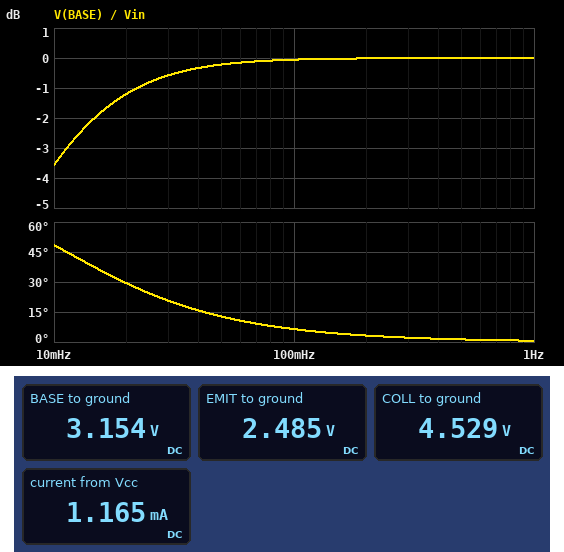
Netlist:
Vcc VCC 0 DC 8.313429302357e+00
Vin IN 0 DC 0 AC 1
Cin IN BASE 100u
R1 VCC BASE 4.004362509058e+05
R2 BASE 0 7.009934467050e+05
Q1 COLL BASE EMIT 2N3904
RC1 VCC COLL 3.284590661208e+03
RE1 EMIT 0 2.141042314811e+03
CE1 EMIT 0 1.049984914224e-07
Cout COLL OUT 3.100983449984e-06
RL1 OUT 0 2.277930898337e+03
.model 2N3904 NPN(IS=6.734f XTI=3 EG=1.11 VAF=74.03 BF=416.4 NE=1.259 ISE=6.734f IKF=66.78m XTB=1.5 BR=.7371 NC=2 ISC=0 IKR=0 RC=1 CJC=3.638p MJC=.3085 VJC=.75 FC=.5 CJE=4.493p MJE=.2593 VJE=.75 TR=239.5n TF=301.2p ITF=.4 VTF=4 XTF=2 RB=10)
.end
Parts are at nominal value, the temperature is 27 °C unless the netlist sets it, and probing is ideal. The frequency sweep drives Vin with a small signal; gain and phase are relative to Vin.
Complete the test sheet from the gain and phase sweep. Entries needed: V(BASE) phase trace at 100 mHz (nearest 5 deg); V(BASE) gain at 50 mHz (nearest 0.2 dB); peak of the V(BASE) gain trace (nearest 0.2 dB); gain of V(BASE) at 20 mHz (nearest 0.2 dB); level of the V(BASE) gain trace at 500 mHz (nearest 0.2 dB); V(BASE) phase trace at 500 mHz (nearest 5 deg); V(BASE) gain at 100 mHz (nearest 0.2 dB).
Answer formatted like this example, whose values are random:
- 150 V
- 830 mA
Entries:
- 5 deg
- -0.2 dB
- 0 dB
- -1.2 dB
- 0 dB
- 0 deg
- 0 dB
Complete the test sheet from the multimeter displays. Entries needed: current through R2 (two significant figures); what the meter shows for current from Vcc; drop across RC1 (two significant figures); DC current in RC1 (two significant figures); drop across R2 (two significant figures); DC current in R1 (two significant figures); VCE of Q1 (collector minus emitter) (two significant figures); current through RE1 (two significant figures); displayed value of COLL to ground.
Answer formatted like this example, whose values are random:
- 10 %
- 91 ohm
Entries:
- 4.5 µA
- 1.165 mA
- 3.8 V
- 1.2 mA
- 3.2 V
- 13 µA
- 2.0 V
- 1.2 mA
- 4.529 V
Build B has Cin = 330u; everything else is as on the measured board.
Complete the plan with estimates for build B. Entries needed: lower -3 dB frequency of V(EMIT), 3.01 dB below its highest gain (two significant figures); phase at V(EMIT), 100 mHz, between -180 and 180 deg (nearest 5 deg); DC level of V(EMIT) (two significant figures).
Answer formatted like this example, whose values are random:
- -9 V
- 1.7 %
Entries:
- 3.4 mHz
- 0 deg
- 2.5 V
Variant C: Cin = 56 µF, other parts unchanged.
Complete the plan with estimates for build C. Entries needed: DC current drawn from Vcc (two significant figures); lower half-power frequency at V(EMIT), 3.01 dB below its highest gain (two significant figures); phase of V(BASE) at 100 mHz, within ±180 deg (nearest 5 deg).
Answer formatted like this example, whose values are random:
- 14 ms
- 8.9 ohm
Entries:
- 1.2 mA
- 20 mHz
- 10 deg
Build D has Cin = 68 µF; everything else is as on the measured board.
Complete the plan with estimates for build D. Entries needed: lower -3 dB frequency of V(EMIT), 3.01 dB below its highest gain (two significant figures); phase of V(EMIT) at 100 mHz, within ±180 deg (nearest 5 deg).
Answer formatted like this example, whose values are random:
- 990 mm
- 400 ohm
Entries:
- 17 mHz
- 10 deg
